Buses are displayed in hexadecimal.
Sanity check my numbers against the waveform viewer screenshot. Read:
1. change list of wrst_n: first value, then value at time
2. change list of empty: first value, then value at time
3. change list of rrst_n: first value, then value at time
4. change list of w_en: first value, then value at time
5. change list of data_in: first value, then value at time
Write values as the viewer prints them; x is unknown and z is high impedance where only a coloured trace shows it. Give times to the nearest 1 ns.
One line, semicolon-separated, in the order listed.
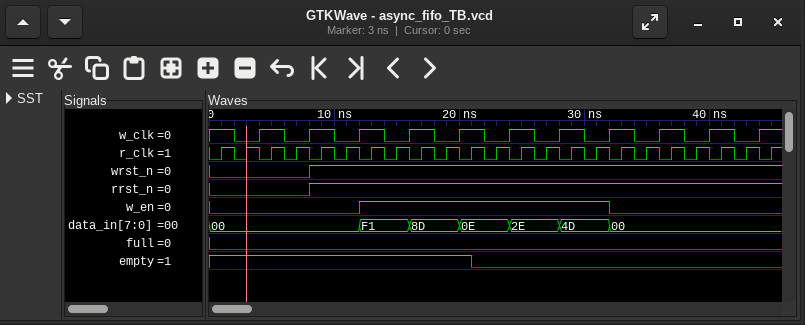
0, 1 at 8 ns; 1, 0 at 21 ns; 0, 1 at 8 ns; 0, 1 at 12 ns, 0 at 32 ns; 00, F1 at 12 ns, 8D at 16 ns, 0E at 20 ns, 2E at 24 ns, 4D at 28 ns, 00 at 32 ns
